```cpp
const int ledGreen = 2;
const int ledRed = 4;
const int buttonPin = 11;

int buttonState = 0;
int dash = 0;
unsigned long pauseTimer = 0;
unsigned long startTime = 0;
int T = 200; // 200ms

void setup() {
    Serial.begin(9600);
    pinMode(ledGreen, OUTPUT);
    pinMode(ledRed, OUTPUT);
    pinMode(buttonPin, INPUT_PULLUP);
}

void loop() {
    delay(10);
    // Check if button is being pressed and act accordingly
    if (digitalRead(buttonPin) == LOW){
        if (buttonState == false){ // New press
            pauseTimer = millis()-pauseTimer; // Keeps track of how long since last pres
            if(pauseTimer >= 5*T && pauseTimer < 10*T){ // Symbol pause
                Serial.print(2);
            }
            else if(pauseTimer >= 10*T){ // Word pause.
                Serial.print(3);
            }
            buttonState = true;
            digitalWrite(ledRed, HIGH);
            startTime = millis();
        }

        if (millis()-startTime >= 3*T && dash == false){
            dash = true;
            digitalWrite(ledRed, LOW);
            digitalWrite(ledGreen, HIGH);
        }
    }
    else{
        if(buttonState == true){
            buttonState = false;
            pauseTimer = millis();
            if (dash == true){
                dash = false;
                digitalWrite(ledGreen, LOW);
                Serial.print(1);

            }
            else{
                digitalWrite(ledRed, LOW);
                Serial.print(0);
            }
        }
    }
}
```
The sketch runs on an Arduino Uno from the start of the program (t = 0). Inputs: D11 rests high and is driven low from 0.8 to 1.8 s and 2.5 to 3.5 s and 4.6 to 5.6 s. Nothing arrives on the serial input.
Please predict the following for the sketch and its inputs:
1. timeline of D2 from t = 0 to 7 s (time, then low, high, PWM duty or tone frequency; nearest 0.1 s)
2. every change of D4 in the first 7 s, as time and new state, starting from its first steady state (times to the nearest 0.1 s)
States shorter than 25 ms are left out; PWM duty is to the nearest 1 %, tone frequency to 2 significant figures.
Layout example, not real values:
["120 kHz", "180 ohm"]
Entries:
["0 s low; 1.4 s high; 1.8 s low; 3.1 s high; 3.5 s low; 5.2 s high; 5.6 s low", "0 s low; 0.8 s high; 1.4 s low; 2.5 s high; 3.1 s low; 4.6 s high; 5.2 s low"]
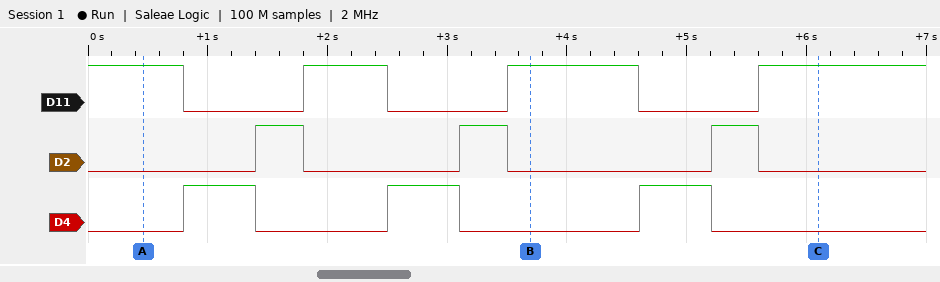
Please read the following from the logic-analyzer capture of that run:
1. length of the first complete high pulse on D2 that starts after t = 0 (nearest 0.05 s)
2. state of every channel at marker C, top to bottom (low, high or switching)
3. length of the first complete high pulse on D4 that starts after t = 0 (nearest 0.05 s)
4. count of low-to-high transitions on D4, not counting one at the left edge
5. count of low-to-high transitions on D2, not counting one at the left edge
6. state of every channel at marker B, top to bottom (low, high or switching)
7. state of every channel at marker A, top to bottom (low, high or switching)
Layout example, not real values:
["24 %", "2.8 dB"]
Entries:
["0.40 s", "D11 high, D2 low, D4 low", "0.60 s", "3", "3", "D11 high, D2 low, D4 low", "D11 high, D2 low, D4 low"]
